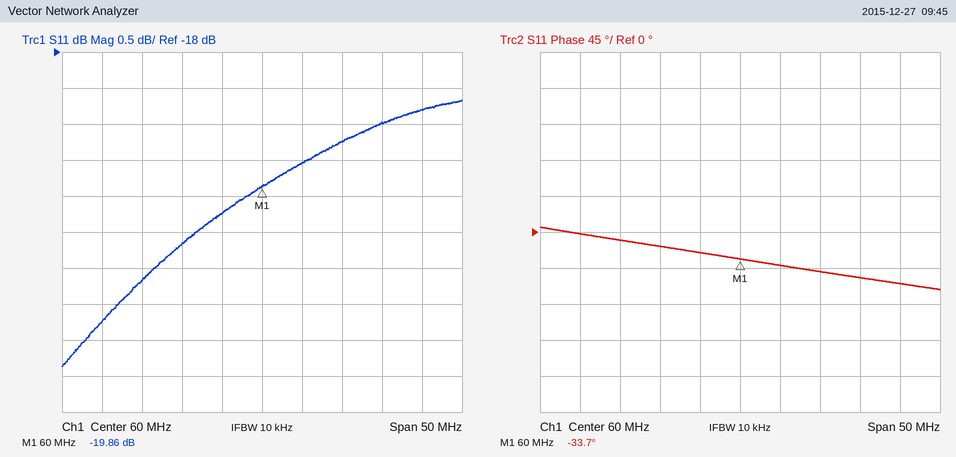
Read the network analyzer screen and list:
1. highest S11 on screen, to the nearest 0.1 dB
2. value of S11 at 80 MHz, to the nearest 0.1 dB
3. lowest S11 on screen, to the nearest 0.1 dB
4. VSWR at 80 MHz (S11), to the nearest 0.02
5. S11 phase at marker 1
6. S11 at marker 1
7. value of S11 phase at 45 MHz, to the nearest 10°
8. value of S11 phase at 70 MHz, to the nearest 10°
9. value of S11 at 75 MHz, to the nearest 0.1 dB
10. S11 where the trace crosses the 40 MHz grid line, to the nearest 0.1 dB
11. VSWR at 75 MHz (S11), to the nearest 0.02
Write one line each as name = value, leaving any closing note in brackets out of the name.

highest S11 on screen, to the nearest 0.1 dB = -18.7 dB
value of S11 at 80 MHz, to the nearest 0.1 dB = -18.8 dB
lowest S11 on screen, to the nearest 0.1 dB = -22.4 dB
VSWR at 80 MHz (S11), to the nearest 0.02 = 1.26
S11 phase at marker 1 = -33.7°
S11 at marker 1 = -19.86 dB
value of S11 phase at 45 MHz, to the nearest 10° = -10°
value of S11 phase at 70 MHz, to the nearest 10° = -50°
value of S11 at 75 MHz, to the nearest 0.1 dB = -19.0 dB
S11 where the trace crosses the 40 MHz grid line, to the nearest 0.1 dB = -21.7 dB
VSWR at 75 MHz (S11), to the nearest 0.02 = 1.26
